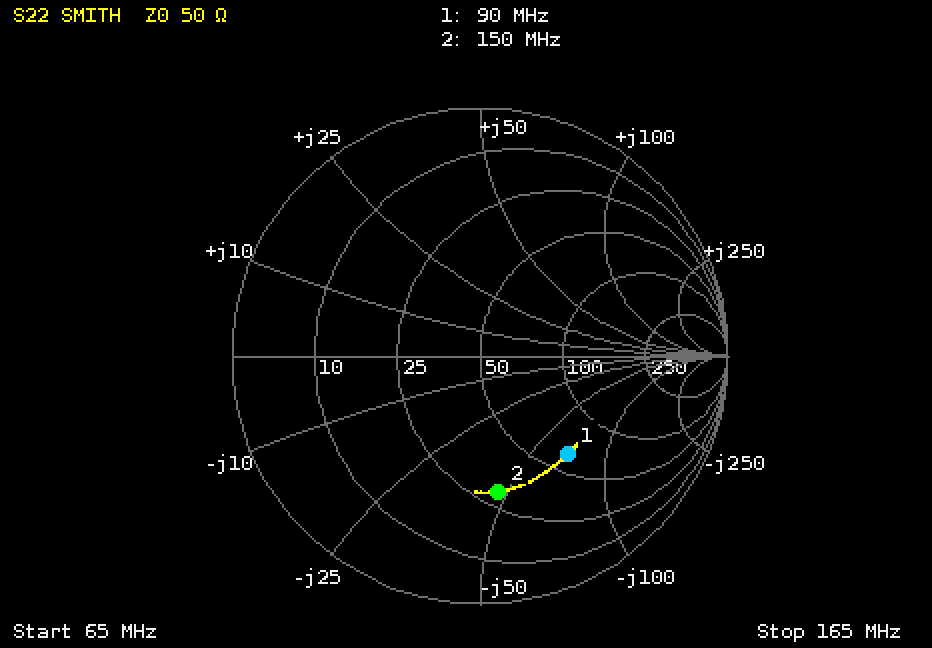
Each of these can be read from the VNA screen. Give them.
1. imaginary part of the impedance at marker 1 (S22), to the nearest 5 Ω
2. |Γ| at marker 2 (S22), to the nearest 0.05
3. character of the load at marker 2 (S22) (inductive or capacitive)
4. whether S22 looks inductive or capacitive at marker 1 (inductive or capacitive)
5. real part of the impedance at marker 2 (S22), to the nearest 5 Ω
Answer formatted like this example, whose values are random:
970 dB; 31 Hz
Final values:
-70 Ω; 0.55; capacitive; capacitive; 30 Ω
